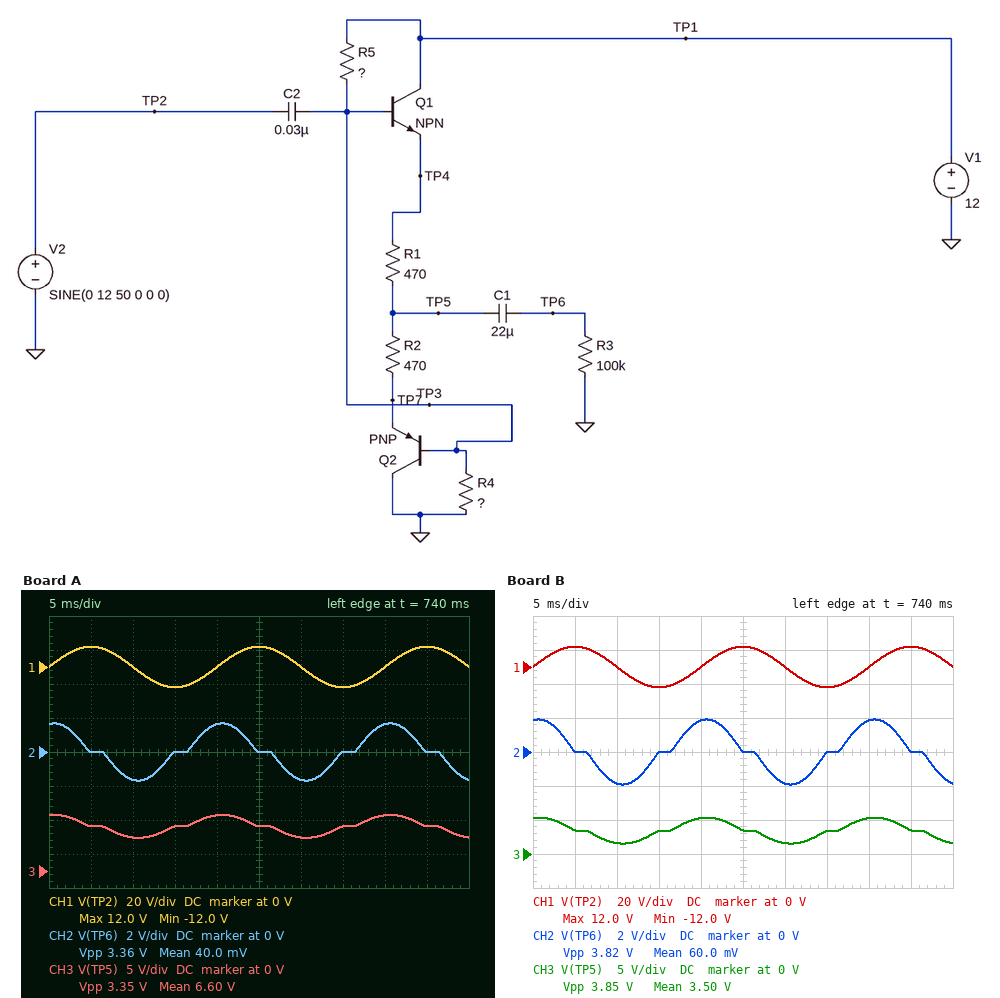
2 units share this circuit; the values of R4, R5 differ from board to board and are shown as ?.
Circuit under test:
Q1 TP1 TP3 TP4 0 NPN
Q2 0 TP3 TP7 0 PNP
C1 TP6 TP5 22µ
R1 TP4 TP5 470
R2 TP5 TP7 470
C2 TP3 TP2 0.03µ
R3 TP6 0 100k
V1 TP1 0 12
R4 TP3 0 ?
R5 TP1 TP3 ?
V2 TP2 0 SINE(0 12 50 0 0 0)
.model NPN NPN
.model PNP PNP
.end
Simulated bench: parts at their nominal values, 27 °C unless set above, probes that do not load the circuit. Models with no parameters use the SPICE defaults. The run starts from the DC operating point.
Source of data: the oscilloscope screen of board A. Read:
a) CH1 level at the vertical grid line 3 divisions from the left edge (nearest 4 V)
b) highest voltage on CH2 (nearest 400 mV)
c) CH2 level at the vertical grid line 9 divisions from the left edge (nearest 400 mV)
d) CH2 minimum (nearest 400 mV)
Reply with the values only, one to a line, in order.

-12 V
1.6 V
0 V
-1.6 V
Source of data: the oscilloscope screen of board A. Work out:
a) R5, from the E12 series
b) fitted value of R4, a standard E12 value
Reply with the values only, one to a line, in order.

39 kΩ
47 kΩ
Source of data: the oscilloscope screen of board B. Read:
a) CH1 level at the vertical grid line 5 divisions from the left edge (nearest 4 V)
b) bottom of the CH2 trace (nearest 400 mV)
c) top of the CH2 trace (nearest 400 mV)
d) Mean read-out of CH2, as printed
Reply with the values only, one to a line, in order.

12 V
-2.0 V
2.0 V
60.0 mV
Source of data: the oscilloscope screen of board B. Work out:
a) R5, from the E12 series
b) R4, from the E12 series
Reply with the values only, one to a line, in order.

82 kΩ
33 kΩ
